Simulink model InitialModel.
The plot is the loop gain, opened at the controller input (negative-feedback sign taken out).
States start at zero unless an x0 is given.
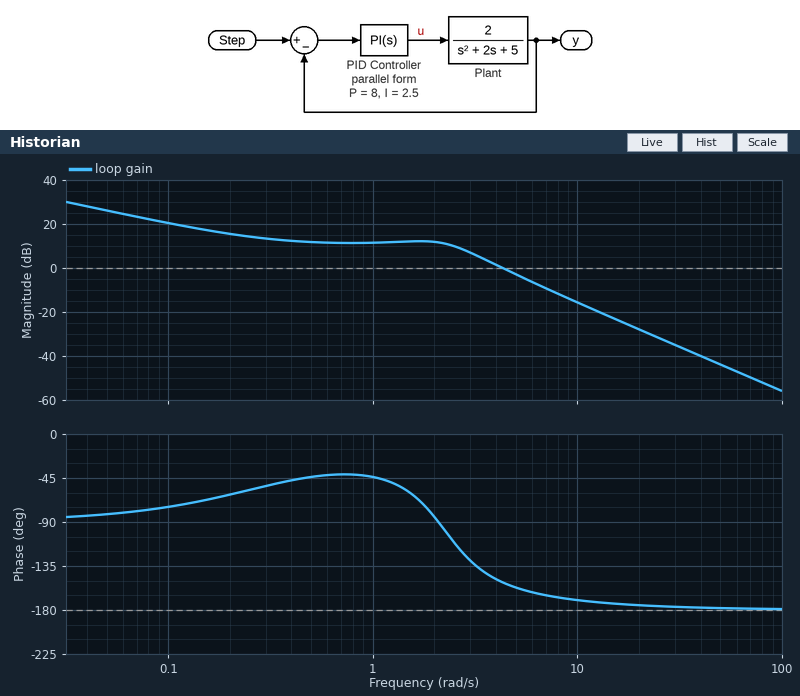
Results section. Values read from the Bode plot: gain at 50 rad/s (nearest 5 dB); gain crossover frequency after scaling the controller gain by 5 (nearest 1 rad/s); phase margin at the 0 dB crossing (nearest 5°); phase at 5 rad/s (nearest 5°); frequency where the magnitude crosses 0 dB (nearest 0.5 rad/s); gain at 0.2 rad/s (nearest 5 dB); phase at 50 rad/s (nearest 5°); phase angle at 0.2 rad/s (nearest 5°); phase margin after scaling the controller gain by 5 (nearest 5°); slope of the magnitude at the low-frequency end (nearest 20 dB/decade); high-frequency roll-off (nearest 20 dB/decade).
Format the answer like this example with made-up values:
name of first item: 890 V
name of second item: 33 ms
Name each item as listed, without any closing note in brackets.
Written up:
gain at 50 rad/s: -45 dB
gain crossover frequency after scaling the controller gain by 5: 9 rad/s
phase margin at the 0 dB crossing: 30°
phase at 5 rad/s: -155°
frequency where the magnitude crosses 0 dB: 4.5 rad/s
gain at 0.2 rad/s: 15 dB
phase at 50 rad/s: -180°
phase angle at 0.2 rad/s: -60°
phase margin after scaling the controller gain by 5: 10°
slope of the magnitude at the low-frequency end: -20 dB/decade
high-frequency roll-off: -40 dB/decade
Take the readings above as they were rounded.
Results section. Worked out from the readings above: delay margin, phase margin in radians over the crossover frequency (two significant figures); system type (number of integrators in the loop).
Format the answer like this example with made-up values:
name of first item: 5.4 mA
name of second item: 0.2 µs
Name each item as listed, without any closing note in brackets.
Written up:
delay margin, phase margin in radians over the crossover frequency: 0.12 s
system type: 1
